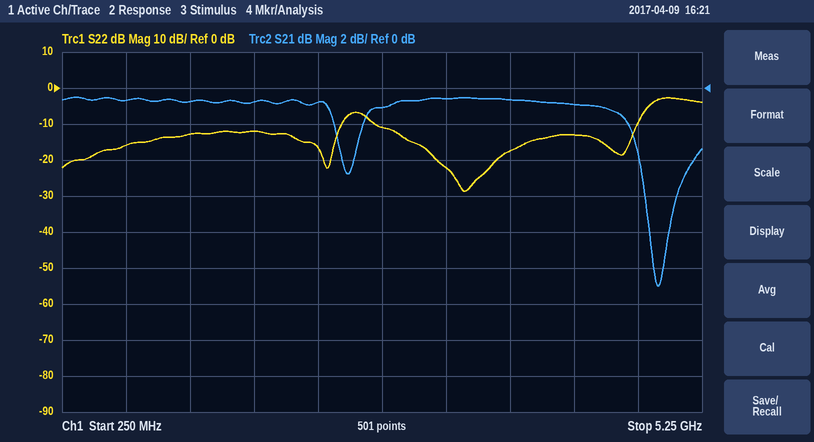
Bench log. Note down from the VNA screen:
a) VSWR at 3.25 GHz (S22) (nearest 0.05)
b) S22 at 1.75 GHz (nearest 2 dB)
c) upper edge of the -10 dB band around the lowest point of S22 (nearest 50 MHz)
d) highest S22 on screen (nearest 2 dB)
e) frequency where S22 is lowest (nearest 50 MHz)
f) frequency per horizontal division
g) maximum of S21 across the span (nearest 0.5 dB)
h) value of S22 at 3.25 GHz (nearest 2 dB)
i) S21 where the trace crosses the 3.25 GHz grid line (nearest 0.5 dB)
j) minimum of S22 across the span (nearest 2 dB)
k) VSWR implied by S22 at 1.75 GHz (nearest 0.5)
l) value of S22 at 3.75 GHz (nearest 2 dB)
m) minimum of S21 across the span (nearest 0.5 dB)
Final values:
1.15
-12 dB
4.75 GHz
-2 dB
3.40 GHz
500 MHz
-0.5 dB
-22 dB
-0.5 dB
-28 dB
1.5
-18 dB
-11.0 dB
